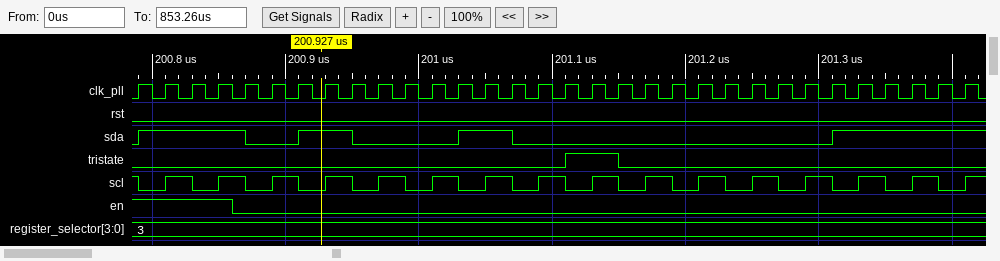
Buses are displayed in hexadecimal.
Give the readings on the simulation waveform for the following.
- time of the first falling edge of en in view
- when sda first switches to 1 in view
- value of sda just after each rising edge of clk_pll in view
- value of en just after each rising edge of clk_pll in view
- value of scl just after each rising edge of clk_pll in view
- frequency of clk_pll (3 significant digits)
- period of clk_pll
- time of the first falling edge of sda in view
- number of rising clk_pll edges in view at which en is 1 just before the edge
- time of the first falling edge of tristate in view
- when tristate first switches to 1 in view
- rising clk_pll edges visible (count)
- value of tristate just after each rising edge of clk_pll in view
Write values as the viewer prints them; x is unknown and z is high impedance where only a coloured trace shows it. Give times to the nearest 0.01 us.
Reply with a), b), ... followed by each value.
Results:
a) 200.86 us
b) 200.79 us
c) 1 1 1 1 0 0 1 1 0 0 0 0 1 1 0 0 0 0 0 0 0 0 0 0 0 0 1 1 1 1 1 1
d) 1 1 1 1 0 0 0 0 0 0 0 0 0 0 0 0 0 0 0 0 0 0 0 0 0 0 0 0 0 0 0 0
e) 0 1 0 1 0 1 0 1 0 1 0 1 0 1 0 1 0 1 0 1 0 1 0 1 0 1 0 1 0 1 0 1
f) 50.0 MHz
g) 0.02 us
h) 200.87 us
i) 4
j) 201.15 us
k) 201.11 us
l) 32
m) 0 0 0 0 0 0 0 0 0 0 0 0 0 0 0 0 1 1 0 0 0 0 0 0 0 0 0 0 0 0 0 0
